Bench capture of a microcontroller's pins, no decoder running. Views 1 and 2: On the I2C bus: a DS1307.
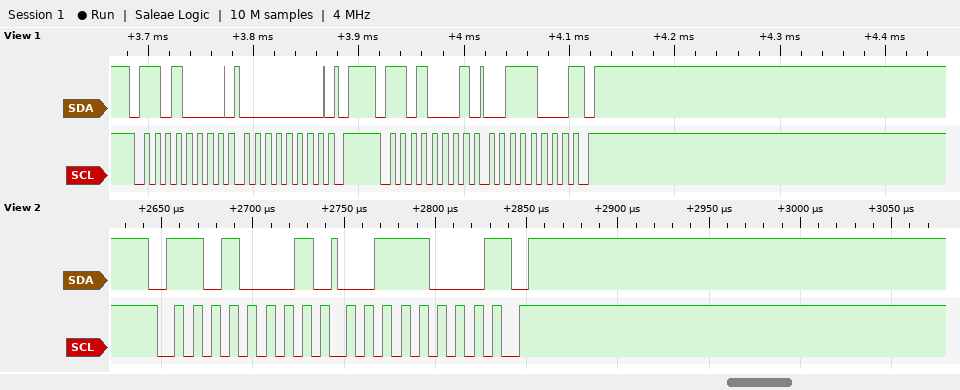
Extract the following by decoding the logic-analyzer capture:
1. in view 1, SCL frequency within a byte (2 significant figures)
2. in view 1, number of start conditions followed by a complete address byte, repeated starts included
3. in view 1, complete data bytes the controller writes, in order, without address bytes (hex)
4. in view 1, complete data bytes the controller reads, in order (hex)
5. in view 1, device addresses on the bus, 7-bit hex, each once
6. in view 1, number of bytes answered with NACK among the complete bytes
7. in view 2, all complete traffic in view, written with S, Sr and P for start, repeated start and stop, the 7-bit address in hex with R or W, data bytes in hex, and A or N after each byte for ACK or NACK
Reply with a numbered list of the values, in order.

1. 100 kHz
2. 2
3. 00
4. 38
5. 0x68
6. 1
7. S 68R A 38 N P
